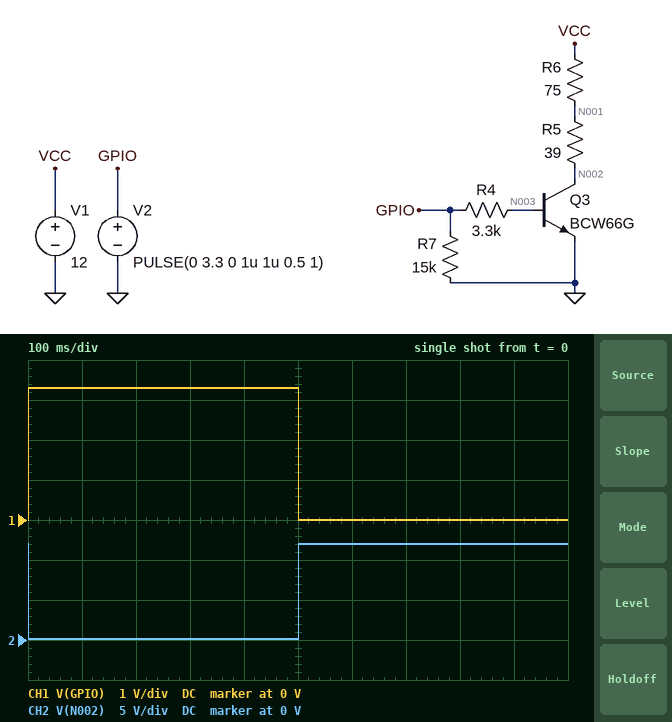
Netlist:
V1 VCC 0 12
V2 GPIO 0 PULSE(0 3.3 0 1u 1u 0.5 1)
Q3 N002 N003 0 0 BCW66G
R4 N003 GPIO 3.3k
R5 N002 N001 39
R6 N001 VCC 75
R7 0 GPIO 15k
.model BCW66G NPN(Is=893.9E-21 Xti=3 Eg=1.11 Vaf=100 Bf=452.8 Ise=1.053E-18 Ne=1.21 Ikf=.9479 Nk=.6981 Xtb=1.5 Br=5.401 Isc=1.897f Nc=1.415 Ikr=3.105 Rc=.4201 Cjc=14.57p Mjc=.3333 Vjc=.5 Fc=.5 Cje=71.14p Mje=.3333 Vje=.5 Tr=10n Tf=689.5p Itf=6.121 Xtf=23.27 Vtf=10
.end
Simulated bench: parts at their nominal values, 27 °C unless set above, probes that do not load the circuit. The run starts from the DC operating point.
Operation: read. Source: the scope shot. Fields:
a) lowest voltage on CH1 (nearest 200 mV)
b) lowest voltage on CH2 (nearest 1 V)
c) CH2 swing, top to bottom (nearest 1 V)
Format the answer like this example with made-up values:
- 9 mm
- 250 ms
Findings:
- 0 V
- 0 V
- 12 V
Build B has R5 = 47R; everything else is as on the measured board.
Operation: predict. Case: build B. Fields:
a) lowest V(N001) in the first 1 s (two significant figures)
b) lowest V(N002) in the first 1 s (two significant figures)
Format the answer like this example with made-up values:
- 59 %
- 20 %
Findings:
- 4.7 V
- 160 mV
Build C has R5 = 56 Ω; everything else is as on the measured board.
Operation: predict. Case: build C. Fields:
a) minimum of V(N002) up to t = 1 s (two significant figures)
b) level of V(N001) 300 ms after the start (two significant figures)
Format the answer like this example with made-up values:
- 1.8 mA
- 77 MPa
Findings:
- 150 mV
- 5.2 V
